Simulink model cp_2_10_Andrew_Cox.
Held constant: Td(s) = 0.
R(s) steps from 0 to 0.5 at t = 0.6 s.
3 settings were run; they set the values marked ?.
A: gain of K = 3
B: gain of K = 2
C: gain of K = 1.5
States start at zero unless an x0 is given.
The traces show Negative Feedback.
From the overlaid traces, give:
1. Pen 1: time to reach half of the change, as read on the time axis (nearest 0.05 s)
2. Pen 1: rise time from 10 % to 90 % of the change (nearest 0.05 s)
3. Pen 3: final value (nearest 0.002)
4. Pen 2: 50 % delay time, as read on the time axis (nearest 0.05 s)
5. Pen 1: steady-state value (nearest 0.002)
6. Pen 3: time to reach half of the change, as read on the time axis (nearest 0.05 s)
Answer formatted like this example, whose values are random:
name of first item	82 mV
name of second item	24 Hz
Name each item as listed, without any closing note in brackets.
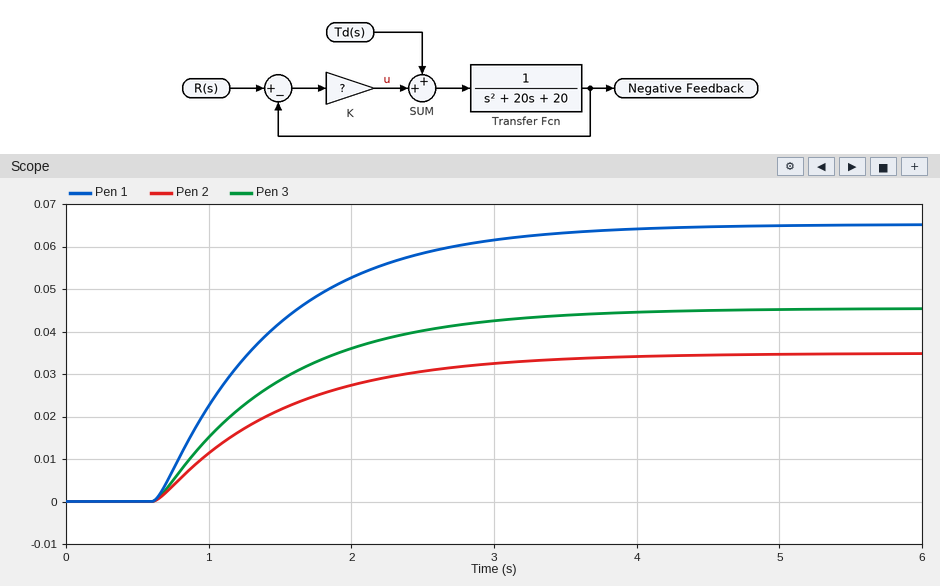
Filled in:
Pen 1: time to reach half of the change, as read on the time axis	1.20 s
Pen 1: rise time from 10 % to 90 % of the change	1.80 s
Pen 3: final value	0.046
Pen 2: 50 % delay time, as read on the time axis	1.25 s
Pen 1: steady-state value	0.066
Pen 3: time to reach half of the change, as read on the time axis	1.25 s
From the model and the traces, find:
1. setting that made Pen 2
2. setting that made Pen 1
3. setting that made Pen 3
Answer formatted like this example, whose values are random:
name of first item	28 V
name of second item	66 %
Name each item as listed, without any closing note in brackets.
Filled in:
setting that made Pen 2	C
setting that made Pen 1	A
setting that made Pen 3	B
